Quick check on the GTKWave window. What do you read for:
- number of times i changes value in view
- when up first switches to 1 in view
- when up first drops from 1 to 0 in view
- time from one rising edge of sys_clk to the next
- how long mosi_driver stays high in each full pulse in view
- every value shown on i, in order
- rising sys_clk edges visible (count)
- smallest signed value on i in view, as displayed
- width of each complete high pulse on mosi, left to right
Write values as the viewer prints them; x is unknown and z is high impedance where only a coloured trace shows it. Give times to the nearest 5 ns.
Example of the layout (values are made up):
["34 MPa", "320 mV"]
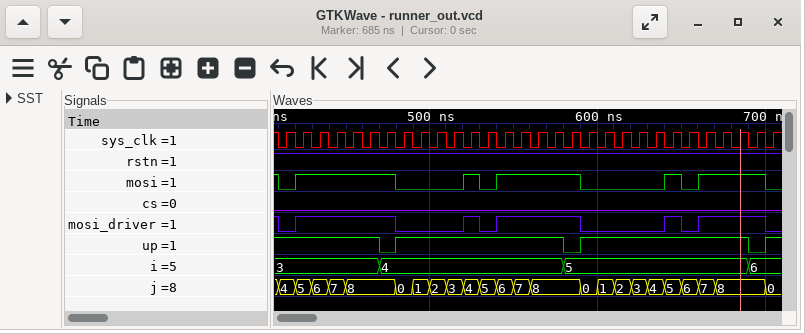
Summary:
["3", "480 ns", "470 ns", "10 ns", "60 ns, 10 ns, 50 ns, 10 ns, 40 ns", "3, 4, 5, 6", "30", "3", "60 ns, 10 ns, 50 ns, 10 ns, 40 ns"]
